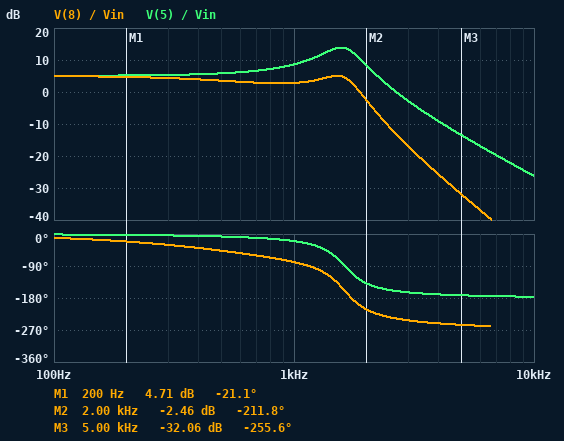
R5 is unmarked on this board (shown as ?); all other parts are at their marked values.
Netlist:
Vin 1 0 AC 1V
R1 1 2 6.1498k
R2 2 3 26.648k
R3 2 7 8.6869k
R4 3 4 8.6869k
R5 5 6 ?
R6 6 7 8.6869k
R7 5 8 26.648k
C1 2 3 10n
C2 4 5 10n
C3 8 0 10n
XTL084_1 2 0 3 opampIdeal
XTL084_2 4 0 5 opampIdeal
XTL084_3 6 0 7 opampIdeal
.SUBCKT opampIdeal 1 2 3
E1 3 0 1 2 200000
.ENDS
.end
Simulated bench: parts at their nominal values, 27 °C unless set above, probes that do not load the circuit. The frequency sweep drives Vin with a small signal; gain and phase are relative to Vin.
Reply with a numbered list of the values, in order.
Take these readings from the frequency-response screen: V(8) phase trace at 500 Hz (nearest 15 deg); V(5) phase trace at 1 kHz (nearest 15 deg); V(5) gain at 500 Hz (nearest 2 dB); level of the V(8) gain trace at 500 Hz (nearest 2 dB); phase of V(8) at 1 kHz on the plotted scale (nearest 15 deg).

1. -45 deg
2. -15 deg
3. 6 dB
4. 4 dB
5. -75 deg
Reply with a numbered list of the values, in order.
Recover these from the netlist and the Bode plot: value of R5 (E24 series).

1. 11 kΩ
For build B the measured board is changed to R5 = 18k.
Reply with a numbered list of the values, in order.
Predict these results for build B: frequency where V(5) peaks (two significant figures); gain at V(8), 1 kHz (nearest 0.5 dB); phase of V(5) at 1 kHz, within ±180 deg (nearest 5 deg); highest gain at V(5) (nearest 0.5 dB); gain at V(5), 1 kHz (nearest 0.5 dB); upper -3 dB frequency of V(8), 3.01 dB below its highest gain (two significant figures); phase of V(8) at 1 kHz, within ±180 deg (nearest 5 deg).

1. 1.2 kHz
2. 9.0 dB
3. -45 deg
4. 16.0 dB
5. 15.0 dB
6. 1.4 kHz
7. -105 deg
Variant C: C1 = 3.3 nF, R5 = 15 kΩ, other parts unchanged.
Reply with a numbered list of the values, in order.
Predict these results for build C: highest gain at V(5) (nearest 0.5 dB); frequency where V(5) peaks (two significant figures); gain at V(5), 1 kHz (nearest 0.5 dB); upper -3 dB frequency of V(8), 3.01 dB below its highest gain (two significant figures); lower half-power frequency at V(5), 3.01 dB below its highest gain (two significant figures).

1. 11.0 dB
2. 2.1 kHz
3. 9.0 dB
4. 660 Hz
5. 420 Hz
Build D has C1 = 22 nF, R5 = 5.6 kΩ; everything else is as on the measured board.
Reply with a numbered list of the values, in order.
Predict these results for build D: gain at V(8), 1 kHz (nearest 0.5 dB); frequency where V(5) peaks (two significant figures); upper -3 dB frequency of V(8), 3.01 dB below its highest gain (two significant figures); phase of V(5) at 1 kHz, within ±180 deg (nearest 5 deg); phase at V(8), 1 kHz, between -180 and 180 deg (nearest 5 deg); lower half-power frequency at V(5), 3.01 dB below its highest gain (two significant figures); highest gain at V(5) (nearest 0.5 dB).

1. -2.0 dB
2. 1.5 kHz
3. 1.6 kHz
4. -10 deg
5. -70 deg
6. 1.4 kHz
7. 14.5 dB
